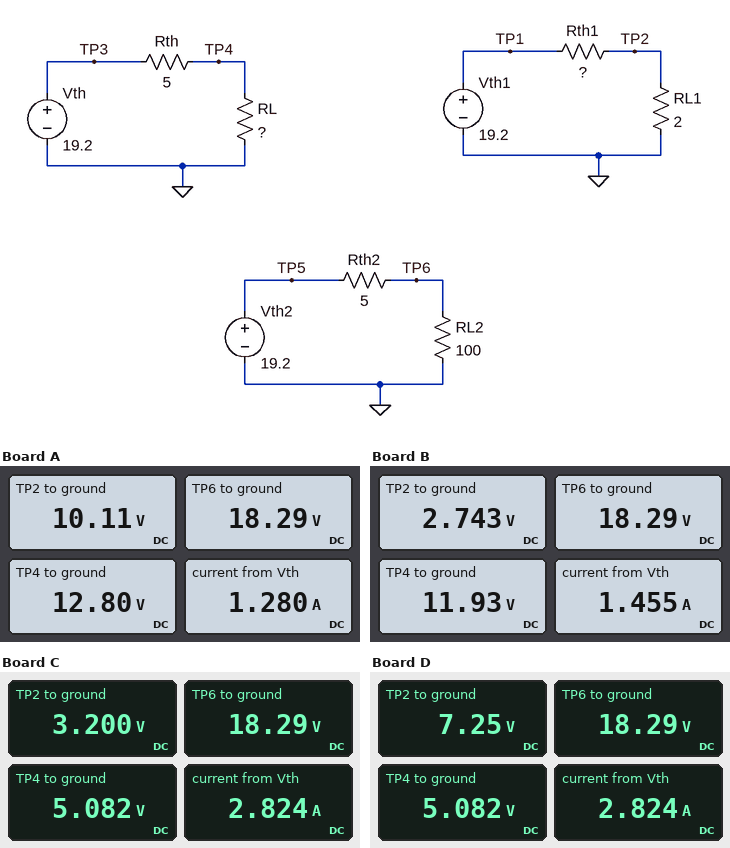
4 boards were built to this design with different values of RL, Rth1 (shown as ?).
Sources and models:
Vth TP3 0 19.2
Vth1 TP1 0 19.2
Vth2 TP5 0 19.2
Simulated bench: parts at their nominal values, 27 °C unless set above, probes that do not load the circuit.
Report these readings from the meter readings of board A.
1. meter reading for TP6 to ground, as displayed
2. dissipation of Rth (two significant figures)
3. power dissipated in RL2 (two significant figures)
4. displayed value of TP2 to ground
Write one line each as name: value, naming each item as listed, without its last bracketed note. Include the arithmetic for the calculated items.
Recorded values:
meter reading for TP6 to ground, as displayed: 18.29 V
dissipation of Rth: (19.2 V - 12.8 V)^2 / 5 Ω = 8.2 W
power dissipated in RL2: (18.29 V)^2 / 100 Ω = 3.3 W
displayed value of TP2 to ground: 10.11 V
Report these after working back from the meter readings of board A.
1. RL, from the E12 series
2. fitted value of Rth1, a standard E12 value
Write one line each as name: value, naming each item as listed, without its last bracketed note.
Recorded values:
RL, from the E12 series: 10 Ω
fitted value of Rth1, a standard E12 value: 1.8 Ω
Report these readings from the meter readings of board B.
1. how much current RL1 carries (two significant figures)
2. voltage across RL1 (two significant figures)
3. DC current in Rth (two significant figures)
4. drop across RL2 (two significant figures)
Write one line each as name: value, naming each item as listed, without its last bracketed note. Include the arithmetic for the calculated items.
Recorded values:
how much current RL1 carries: (2.743 V) / 2 Ω = 1.4 A
voltage across RL1: 2.743 V = 2.7 V
DC current in Rth: (19.2 V - 11.93 V) / 5 Ω = 1.5 A
drop across RL2: 18.29 V = 18 V
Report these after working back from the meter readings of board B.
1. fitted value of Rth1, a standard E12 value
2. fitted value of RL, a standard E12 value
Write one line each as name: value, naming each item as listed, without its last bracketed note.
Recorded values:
fitted value of Rth1, a standard E12 value: 12 Ω
fitted value of RL, a standard E12 value: 8.2 Ω
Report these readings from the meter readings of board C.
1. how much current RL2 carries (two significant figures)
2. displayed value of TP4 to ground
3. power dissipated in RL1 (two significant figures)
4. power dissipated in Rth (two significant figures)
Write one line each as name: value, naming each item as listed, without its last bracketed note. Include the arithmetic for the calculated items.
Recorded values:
how much current RL2 carries: (18.29 V) / 100 Ω = 180 mA
displayed value of TP4 to ground: 5.082 V
power dissipated in RL1: (3.2 V)^2 / 2 Ω = 5.1 W
power dissipated in Rth: (19.2 V - 5.082 V)^2 / 5 Ω = 40 W
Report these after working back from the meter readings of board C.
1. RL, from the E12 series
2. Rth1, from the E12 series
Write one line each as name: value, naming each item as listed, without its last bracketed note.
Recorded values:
RL, from the E12 series: 1.8 Ω
Rth1, from the E12 series: 10 Ω
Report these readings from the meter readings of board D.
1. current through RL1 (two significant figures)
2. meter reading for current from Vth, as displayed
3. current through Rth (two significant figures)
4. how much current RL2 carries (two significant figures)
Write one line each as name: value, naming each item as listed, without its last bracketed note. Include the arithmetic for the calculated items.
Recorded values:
current through RL1: (7.25 V) / 2 Ω = 3.6 A
meter reading for current from Vth, as displayed: 2.824 A
current through Rth: (19.2 V - 5.082 V) / 5 Ω = 2.8 A
how much current RL2 carries: (18.29 V) / 100 Ω = 180 mA
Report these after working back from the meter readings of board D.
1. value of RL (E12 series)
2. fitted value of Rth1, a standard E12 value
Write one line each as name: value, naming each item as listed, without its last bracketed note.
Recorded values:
value of RL: 1.8 Ω
fitted value of Rth1, a standard E12 value: 3.3 Ω
